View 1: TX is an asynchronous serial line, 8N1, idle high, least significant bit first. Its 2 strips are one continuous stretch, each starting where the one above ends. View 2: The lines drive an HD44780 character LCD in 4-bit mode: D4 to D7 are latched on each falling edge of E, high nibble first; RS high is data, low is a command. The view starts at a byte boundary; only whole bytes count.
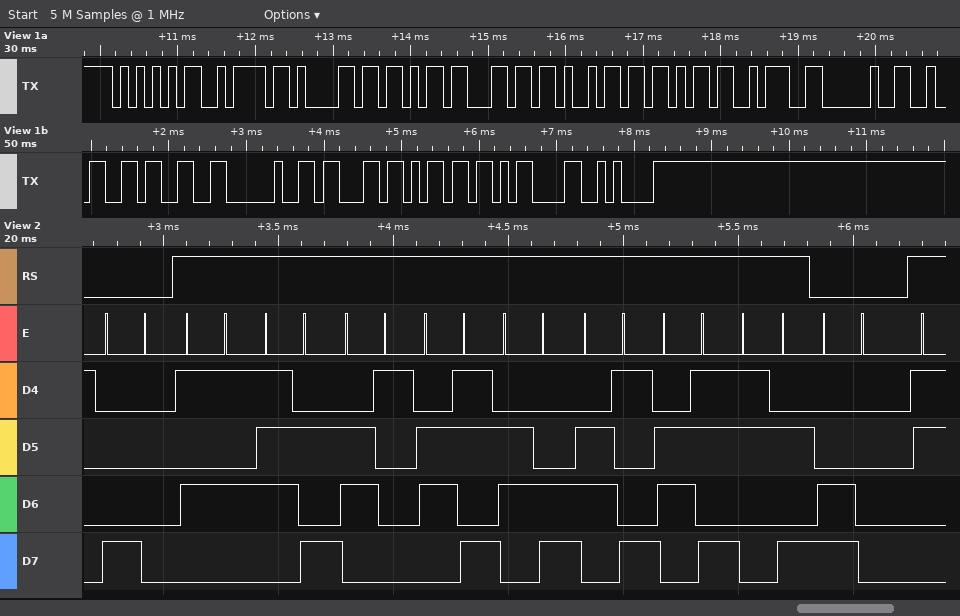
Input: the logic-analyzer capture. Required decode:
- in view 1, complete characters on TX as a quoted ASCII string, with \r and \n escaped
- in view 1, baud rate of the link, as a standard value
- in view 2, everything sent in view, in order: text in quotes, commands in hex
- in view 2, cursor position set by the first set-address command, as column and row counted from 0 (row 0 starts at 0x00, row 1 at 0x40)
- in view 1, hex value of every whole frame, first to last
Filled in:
"Uzaklik: 23 cm\r\n"
9600 baud
0x80 "Uzaklik:" 0xC0
column 0, row 0
55 7A 61 6B 6C 69 6B 3A 20 32 33 20 63 6D 0D 0A
